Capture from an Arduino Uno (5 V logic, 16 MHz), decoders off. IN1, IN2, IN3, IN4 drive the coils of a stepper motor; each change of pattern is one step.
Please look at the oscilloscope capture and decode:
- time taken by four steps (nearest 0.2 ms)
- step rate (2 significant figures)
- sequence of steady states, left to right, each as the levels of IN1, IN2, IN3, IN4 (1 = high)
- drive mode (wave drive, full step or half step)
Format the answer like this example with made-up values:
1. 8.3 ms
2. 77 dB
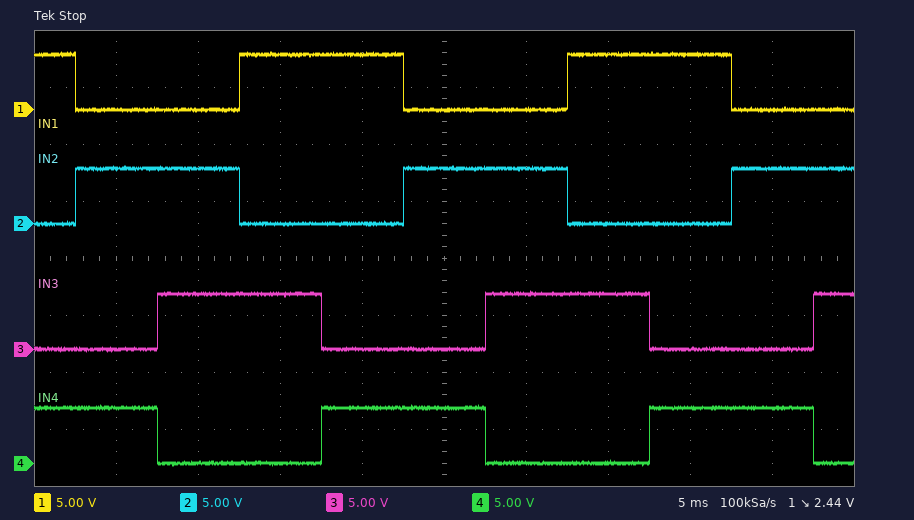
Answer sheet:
1. 20.0 ms
2. 200 steps/s
3. 1001 0101 0110 1010 1001 0101 0110 1010 1001 0101 0110
4. full step
